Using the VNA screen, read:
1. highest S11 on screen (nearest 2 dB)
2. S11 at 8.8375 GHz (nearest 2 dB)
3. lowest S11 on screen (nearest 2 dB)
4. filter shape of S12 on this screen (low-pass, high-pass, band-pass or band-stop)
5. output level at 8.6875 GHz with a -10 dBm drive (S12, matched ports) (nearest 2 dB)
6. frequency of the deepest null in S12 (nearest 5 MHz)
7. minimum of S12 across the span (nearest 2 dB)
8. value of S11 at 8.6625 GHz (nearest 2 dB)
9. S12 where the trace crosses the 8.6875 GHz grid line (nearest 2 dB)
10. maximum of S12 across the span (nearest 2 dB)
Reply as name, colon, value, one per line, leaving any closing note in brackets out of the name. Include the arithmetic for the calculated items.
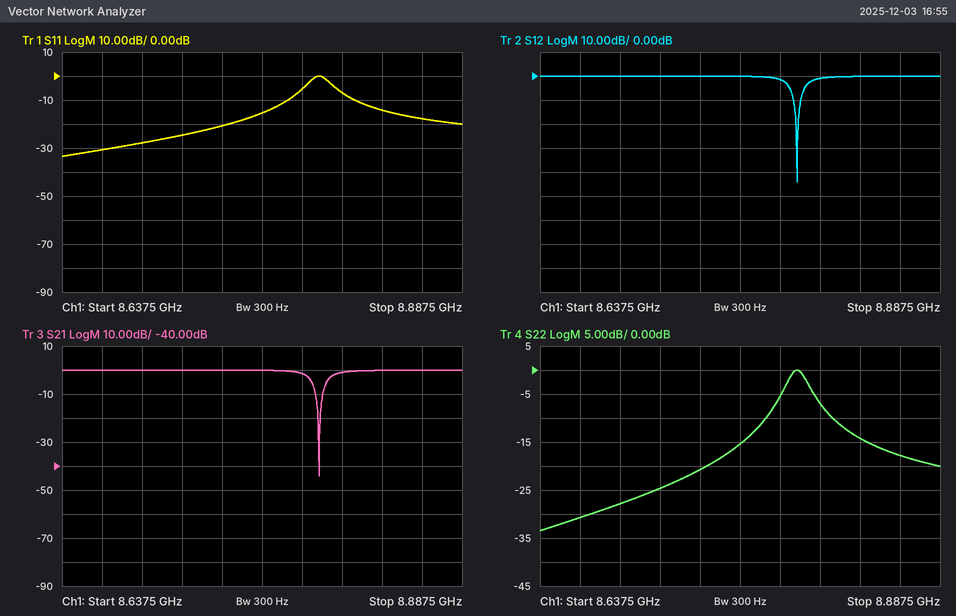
highest S11 on screen: 0 dB
S11 at 8.8375 GHz: -14 dB
lowest S11 on screen: -34 dB
filter shape of S12 on this screen: band-stop
output level at 8.6875 GHz with a -10 dBm drive (S12, matched ports): -10 dBm + (0 dB) = -10 dBm
frequency of the deepest null in S12: 8.800 GHz
minimum of S12 across the span: -44 dB
value of S11 at 8.6625 GHz: -30 dB
S12 where the trace crosses the 8.6875 GHz grid line: 0 dB
maximum of S12 across the span: 0 dB
